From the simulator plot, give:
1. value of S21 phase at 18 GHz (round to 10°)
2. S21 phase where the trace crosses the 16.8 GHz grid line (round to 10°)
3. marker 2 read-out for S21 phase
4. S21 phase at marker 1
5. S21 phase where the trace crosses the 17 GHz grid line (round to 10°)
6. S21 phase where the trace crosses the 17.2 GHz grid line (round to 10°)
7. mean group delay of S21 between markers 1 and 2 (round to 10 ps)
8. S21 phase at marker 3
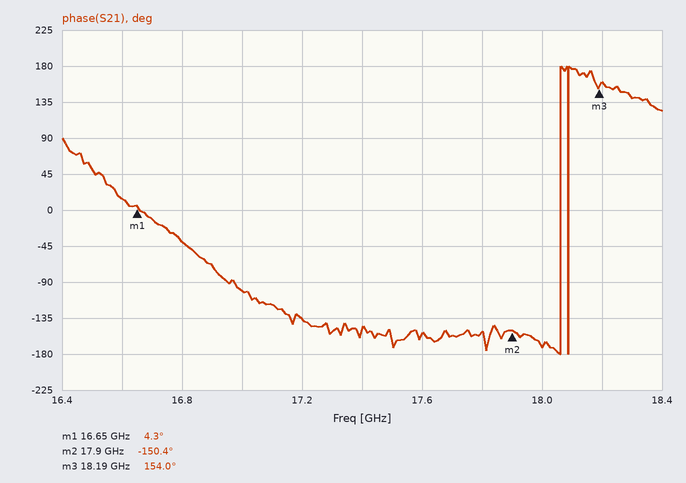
-170°
-40°
-150.4°
4.3°
-100°
-140°
340 ps
154.0°
